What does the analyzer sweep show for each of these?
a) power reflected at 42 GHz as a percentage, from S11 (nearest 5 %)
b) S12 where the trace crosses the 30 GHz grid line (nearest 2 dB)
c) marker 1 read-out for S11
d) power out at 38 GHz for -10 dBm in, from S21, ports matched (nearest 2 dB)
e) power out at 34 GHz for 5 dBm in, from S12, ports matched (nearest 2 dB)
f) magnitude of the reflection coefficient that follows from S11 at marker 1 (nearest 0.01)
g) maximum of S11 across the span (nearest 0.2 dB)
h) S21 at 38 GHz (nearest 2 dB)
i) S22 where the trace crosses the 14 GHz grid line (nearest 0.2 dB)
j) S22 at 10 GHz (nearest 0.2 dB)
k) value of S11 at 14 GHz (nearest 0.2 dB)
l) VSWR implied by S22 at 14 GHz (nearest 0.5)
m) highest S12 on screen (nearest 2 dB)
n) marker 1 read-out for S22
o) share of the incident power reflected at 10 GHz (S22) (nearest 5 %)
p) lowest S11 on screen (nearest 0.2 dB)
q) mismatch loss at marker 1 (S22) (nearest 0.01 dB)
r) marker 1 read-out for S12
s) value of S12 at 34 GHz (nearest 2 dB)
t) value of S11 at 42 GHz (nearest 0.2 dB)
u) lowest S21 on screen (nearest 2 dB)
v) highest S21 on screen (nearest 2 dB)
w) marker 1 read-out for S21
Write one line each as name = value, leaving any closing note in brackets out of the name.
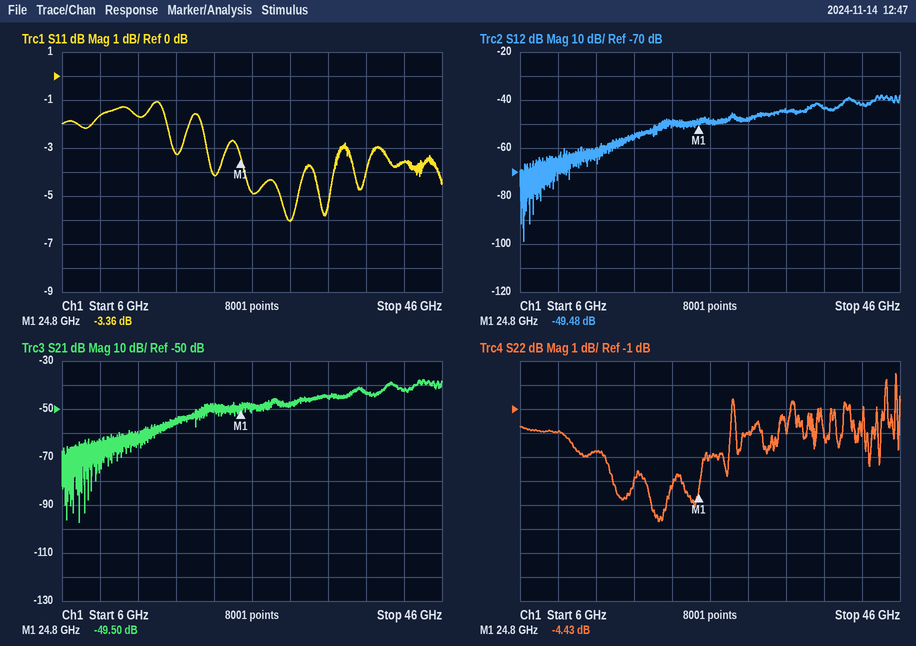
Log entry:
power reflected at 42 GHz as a percentage, from S11 = 45 %
S12 where the trace crosses the 30 GHz grid line = -48 dB
marker 1 read-out for S11 = -3.36 dB
power out at 38 GHz for -10 dBm in, from S21, ports matched = -54 dBm
power out at 34 GHz for 5 dBm in, from S12, ports matched = -40 dBm
magnitude of the reflection coefficient that follows from S11 at marker 1 = 0.68
maximum of S11 across the span = -1.0 dB
S21 at 38 GHz = -44 dB
S22 where the trace crosses the 14 GHz grid line = -2.8 dB
S22 at 10 GHz = -2.0 dB
value of S11 at 14 GHz = -1.6 dB
VSWR implied by S22 at 14 GHz = 6.5
highest S12 on screen = -38 dB
marker 1 read-out for S22 = -4.43 dB
share of the incident power reflected at 10 GHz (S22) = 65 %
lowest S11 on screen = -6.0 dB
mismatch loss at marker 1 (S22) = 1.94 dB
marker 1 read-out for S12 = -49.48 dB
value of S12 at 34 GHz = -44 dB
value of S11 at 42 GHz = -3.6 dB
lowest S21 on screen = -98 dB
highest S21 on screen = -38 dB
marker 1 read-out for S21 = -49.50 dB
